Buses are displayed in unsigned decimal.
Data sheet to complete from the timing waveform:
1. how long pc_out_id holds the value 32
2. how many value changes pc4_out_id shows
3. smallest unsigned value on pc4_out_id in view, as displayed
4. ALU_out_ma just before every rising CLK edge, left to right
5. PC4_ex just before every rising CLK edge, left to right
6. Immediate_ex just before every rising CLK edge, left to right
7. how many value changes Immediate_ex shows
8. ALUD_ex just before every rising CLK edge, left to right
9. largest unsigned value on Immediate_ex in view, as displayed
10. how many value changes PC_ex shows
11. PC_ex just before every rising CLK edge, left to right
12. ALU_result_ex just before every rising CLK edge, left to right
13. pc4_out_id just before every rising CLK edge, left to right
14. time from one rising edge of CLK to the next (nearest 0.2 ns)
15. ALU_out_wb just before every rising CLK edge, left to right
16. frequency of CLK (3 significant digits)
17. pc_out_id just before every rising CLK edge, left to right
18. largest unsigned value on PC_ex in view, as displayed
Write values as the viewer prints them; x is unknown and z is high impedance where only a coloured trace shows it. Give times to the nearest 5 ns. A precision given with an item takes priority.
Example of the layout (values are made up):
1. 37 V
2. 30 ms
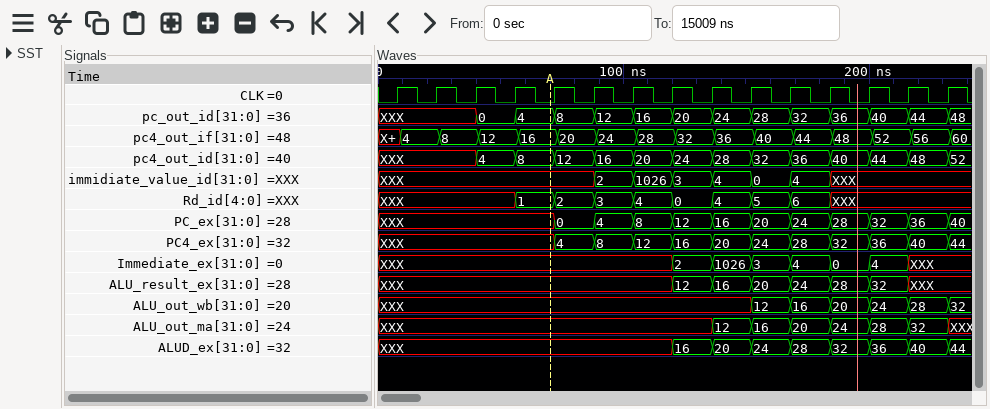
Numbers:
1. 15 ns
2. 13
3. 4
4. XXX, XXX, XXX, XXX, XXX, XXX, XXX, XXX, XXX, 12, 16, 20, 24, 28, 32
5. XXX, XXX, XXX, XXX, XXX, 4, 8, 12, 16, 20, 24, 28, 32, 36, 40
6. XXX, XXX, XXX, XXX, XXX, XXX, XXX, XXX, 2, 1026, 3, 4, 0, 4, XXX
7. 7
8. XXX, XXX, XXX, XXX, XXX, XXX, XXX, XXX, 16, 20, 24, 28, 32, 36, 40
9. 1026
10. 11
11. XXX, XXX, XXX, XXX, XXX, 0, 4, 8, 12, 16, 20, 24, 28, 32, 36
12. XXX, XXX, XXX, XXX, XXX, XXX, XXX, XXX, 12, 16, 20, 24, 28, 32, XXX
13. XXX, XXX, XXX, 4, 8, 12, 16, 20, 24, 28, 32, 36, 40, 44, 48
14. 16 ns
15. XXX, XXX, XXX, XXX, XXX, XXX, XXX, XXX, XXX, XXX, 12, 16, 20, 24, 28
16. 62.5 MHz
17. XXX, XXX, XXX, 0, 4, 8, 12, 16, 20, 24, 28, 32, 36, 40, 44
18. 40
